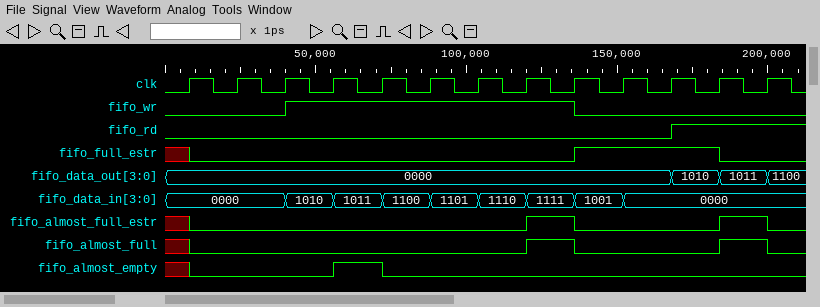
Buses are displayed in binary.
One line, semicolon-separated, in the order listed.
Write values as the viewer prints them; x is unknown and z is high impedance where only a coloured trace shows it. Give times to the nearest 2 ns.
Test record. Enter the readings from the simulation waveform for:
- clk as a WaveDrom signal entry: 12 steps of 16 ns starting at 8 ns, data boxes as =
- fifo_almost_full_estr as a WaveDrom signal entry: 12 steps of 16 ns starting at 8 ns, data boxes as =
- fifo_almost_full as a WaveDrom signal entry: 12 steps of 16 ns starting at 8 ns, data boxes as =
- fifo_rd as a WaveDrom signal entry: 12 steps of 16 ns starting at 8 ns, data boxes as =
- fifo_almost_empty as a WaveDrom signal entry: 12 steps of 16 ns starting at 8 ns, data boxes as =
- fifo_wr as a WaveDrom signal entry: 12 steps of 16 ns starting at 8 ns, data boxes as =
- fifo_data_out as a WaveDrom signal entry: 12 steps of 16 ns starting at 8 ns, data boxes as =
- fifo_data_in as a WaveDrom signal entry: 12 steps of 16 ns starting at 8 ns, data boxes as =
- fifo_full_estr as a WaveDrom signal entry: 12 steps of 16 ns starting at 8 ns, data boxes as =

{name: 'clk', wave: 'p...........'}; {name: 'fifo_almost_full_estr', wave: '0......10..1'}; {name: 'fifo_almost_full', wave: '0......10..1'}; {name: 'fifo_rd', wave: '0.........1.'}; {name: 'fifo_almost_empty', wave: '0..10.......'}; {name: 'fifo_wr', wave: '0.1.....0...'}; {name: 'fifo_data_out', wave: '=.........==', data: '0000 1010 1011'}; {name: 'fifo_data_in', wave: '=.========..', data: '0000 1010 1011 1100 1101 1110 1111 1001 0000'}; {name: 'fifo_full_estr', wave: '0.......1..0'}
